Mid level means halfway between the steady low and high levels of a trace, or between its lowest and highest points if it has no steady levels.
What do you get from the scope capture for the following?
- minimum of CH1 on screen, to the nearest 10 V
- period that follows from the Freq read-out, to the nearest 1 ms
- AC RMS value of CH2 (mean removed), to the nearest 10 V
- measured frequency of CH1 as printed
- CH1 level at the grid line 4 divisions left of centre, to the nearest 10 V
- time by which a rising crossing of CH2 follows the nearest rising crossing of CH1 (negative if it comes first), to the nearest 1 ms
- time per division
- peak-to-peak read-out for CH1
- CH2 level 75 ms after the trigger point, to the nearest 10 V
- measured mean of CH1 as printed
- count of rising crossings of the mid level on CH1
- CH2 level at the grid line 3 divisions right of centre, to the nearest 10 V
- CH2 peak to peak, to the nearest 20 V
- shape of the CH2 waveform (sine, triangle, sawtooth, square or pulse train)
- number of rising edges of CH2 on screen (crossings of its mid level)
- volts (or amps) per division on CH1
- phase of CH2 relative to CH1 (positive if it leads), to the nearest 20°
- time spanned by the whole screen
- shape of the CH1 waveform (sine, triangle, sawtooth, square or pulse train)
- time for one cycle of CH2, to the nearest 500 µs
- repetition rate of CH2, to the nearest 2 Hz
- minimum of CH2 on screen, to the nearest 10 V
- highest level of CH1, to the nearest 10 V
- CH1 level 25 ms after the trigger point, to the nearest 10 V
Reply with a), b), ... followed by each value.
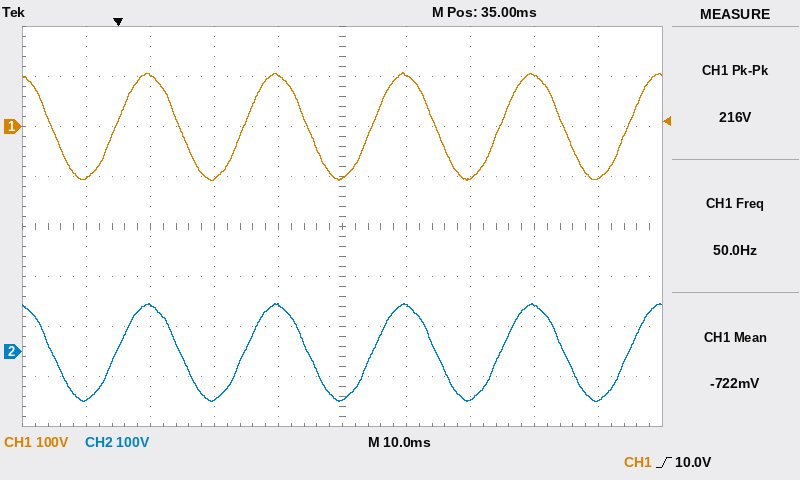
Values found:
a) -110 V
b) 20 ms
c) 70 V
d) 50.0 Hz
e) -100 V
f) 0 ms
g) 10 ms
h) 216 V
i) -100 V
j) -722 mV
k) 5
l) 90 V
m) 200 V
n) sine
o) 5
p) 100 V
q) 0°
r) 100 ms
s) sine
t) 20.0 ms
u) 50 Hz
v) -100 V
w) 110 V
x) 100 V
